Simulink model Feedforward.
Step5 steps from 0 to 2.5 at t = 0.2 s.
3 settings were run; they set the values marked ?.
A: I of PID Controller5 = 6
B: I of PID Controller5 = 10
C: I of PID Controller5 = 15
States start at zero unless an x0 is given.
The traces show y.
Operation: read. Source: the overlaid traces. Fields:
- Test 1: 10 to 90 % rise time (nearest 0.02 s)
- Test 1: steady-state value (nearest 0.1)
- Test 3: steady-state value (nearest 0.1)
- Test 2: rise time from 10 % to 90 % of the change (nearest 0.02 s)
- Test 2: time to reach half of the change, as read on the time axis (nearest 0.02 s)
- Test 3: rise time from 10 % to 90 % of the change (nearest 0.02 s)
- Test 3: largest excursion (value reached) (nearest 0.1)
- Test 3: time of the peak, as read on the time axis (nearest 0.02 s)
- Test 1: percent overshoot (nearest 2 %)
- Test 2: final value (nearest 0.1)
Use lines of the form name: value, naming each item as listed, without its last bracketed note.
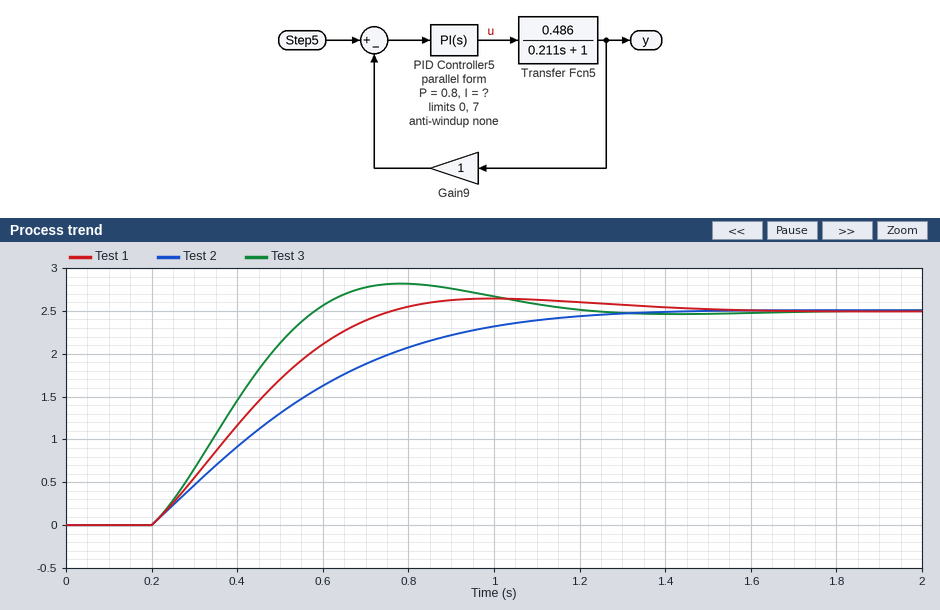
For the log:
Test 1: 10 to 90 % rise time: 0.40 s
Test 1: steady-state value: 2.5
Test 3: steady-state value: 2.5
Test 2: rise time from 10 % to 90 % of the change: 0.68 s
Test 2: time to reach half of the change, as read on the time axis: 0.48 s
Test 3: rise time from 10 % to 90 % of the change: 0.28 s
Test 3: largest excursion (value reached): 2.8
Test 3: time of the peak, as read on the time axis: 0.78 s
Test 1: percent overshoot: 6 %
Test 2: final value: 2.5
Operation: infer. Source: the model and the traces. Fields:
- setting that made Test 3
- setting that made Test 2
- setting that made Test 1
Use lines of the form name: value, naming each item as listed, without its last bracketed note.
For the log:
setting that made Test 3: C
setting that made Test 2: A
setting that made Test 1: B
